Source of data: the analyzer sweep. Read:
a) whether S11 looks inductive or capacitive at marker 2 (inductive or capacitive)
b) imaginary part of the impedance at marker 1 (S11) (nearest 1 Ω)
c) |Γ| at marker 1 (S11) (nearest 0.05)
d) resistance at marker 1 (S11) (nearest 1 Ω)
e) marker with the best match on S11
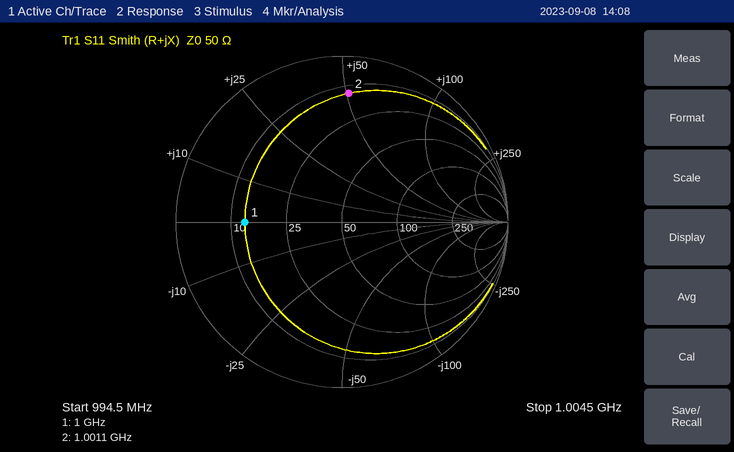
inductive
0 Ω
0.60
13 Ω
marker 1
